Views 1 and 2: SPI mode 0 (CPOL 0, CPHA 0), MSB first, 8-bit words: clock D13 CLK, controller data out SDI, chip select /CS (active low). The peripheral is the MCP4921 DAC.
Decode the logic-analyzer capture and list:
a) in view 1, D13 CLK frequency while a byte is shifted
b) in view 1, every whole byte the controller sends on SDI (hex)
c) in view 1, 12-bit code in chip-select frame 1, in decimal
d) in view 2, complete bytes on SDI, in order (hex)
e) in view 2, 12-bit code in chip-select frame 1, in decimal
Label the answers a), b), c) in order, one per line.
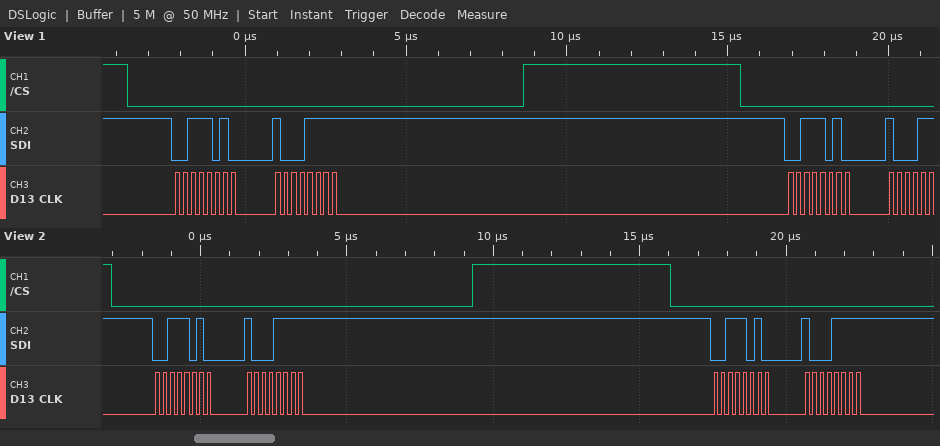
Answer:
a) 4 MHz
b) 3A 8F 3A
c) 2703
d) 3A 8F 3A 8F
e) 2703
